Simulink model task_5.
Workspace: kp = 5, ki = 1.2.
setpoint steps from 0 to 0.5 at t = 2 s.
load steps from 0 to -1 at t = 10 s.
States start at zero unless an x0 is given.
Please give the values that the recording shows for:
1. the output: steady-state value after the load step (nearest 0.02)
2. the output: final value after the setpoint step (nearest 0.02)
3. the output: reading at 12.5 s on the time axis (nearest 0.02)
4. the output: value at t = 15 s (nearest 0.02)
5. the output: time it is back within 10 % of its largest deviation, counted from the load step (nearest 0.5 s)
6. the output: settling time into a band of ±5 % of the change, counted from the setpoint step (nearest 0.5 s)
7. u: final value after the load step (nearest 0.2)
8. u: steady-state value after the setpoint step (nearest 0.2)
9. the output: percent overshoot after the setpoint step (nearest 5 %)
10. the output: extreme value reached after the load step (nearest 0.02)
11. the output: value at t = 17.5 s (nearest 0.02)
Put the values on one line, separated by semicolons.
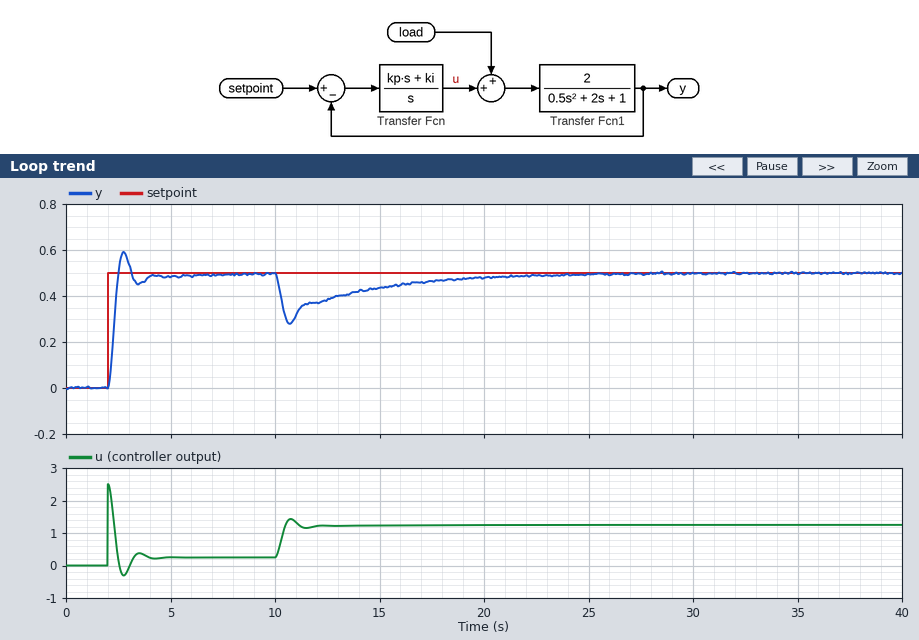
0.50; 0.50; 0.38; 0.44; 10.0 s; 2.0 s; 1.2; 0.2; 20 %; 0.28; 0.46
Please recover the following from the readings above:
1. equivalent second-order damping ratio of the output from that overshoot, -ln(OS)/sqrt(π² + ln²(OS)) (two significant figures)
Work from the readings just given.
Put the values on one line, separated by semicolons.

0.46
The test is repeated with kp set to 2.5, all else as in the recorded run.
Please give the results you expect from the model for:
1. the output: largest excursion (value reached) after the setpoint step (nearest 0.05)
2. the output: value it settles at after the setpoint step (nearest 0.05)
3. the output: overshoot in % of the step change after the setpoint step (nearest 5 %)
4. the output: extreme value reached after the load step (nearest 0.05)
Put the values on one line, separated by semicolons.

0.55; 0.50; 10 %; 0.15
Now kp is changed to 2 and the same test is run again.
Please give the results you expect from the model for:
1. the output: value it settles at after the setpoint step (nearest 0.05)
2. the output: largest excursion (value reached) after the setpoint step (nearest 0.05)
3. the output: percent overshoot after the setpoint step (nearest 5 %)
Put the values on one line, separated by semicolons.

0.50; 0.55; 10 %
